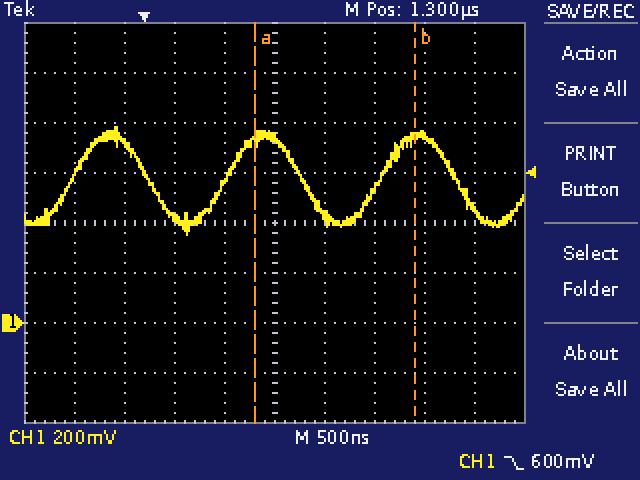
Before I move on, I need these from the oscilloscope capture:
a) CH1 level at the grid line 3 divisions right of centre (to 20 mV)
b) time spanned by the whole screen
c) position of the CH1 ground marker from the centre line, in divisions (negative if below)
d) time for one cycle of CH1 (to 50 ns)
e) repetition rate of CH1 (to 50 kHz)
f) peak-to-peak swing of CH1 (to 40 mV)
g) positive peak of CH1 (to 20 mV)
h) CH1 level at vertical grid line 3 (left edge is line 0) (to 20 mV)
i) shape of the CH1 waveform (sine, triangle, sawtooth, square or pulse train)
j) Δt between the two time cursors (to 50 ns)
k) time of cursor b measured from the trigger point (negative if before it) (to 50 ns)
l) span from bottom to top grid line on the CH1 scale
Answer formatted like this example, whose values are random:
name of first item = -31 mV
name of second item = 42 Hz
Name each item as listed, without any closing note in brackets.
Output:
CH1 level at the grid line 3 divisions right of centre = 740 mV
time spanned by the whole screen = 5 µs
position of the CH1 ground marker from the centre line, in divisions = -2.0 div
time for one cycle of CH1 = 1.55 µs
repetition rate of CH1 = 650 kHz
peak-to-peak swing of CH1 = 440 mV
positive peak of CH1 = 780 mV
CH1 level at vertical grid line 3 (left edge is line 0) = 420 mV
shape of the CH1 waveform = sine
Δt between the two time cursors = 1.60 µs
time of cursor b measured from the trigger point (negative if before it) = +2.70 µs
span from bottom to top grid line on the CH1 scale = 1.6 V
